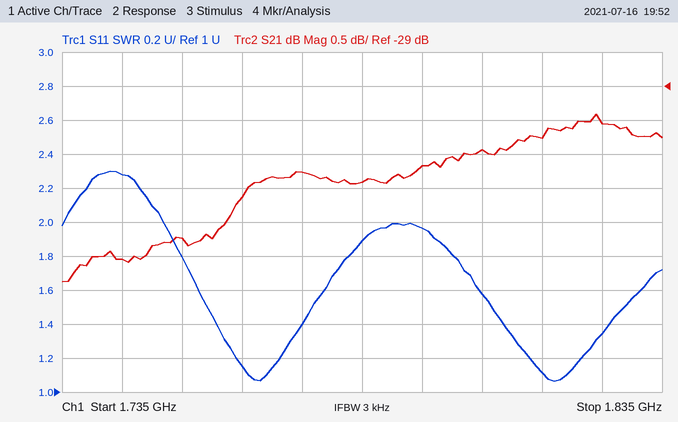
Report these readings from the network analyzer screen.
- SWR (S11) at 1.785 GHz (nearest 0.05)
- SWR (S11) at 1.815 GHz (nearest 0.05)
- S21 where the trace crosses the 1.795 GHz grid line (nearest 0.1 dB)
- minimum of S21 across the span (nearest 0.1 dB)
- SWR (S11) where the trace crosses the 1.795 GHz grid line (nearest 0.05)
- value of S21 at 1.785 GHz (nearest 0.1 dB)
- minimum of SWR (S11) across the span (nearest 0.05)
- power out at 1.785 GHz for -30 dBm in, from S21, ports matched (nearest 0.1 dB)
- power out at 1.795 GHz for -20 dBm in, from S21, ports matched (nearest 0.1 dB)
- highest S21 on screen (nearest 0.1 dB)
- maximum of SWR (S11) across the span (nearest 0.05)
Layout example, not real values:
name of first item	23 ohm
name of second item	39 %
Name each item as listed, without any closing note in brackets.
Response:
SWR (S11) at 1.785 GHz	1.90
SWR (S11) at 1.815 GHz	1.10
S21 where the trace crosses the 1.795 GHz grid line	-30.2 dB
minimum of S21 across the span	-31.9 dB
SWR (S11) where the trace crosses the 1.795 GHz grid line	1.95
value of S21 at 1.785 GHz	-30.4 dB
minimum of SWR (S11) across the span	1.05
power out at 1.785 GHz for -30 dBm in, from S21, ports matched	-60.4 dBm
power out at 1.795 GHz for -20 dBm in, from S21, ports matched	-50.2 dBm
highest S21 on screen	-29.4 dB
maximum of SWR (S11) across the span	2.30
